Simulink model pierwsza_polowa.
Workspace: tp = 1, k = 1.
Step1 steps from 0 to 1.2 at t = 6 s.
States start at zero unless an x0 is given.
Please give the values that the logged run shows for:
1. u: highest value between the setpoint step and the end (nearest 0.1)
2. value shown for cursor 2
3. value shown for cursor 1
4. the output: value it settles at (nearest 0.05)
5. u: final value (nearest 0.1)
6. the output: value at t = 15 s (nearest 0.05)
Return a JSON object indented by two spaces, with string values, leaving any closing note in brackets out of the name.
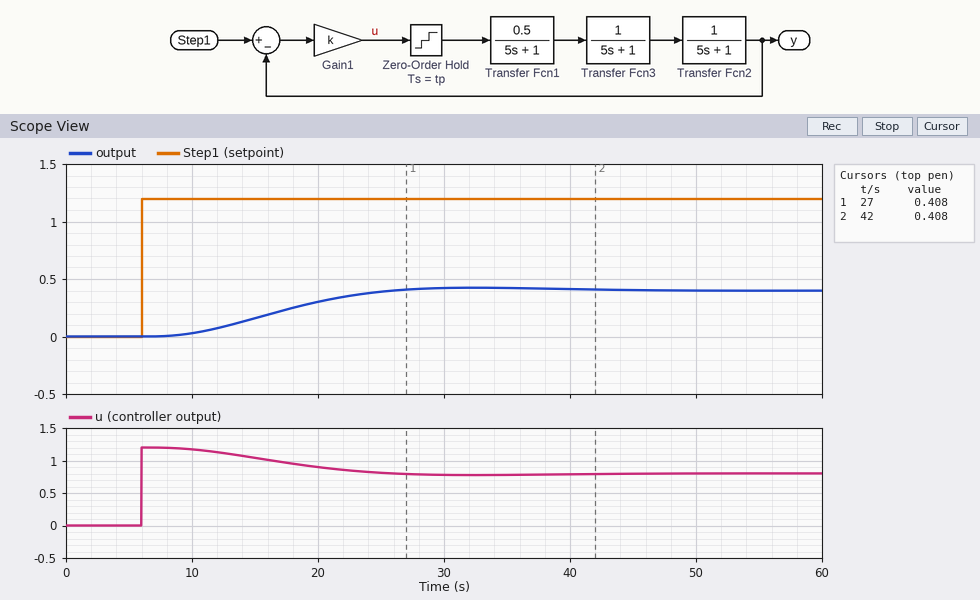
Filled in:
{
  "u: highest value between the setpoint step and the end": "1.2",
  "value shown for cursor 2": "0.408",
  "value shown for cursor 1": "0.408",
  "the output: value it settles at": "0.40",
  "u: final value": "0.8",
  "the output: value at t = 15 s": "0.15"
}
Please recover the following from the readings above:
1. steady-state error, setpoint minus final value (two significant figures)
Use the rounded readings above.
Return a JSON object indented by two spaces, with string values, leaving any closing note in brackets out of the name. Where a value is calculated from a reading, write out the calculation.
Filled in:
{
  "steady-state error, setpoint minus final value": "1.2 - 0.4 = 0.80"
}
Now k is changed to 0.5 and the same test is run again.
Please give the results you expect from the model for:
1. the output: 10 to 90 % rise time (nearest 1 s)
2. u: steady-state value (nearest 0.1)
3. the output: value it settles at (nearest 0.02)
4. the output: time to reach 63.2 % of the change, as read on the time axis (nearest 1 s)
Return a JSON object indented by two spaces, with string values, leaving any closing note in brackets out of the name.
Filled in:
{
  "the output: 10 to 90 % rise time": "15 s",
  "u: steady-state value": "0.5",
  "the output: value it settles at": "0.24",
  "the output: time to reach 63.2 % of the change, as read on the time axis": "20 s"
}
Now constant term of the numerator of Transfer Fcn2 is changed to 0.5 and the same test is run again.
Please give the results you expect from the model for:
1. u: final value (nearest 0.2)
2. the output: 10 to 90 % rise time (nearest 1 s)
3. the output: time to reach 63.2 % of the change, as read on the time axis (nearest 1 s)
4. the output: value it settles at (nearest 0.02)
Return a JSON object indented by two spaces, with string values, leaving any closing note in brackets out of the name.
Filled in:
{
  "u: final value": "1.0",
  "the output: 10 to 90 % rise time": "15 s",
  "the output: time to reach 63.2 % of the change, as read on the time axis": "20 s",
  "the output: value it settles at": "0.24"
}
